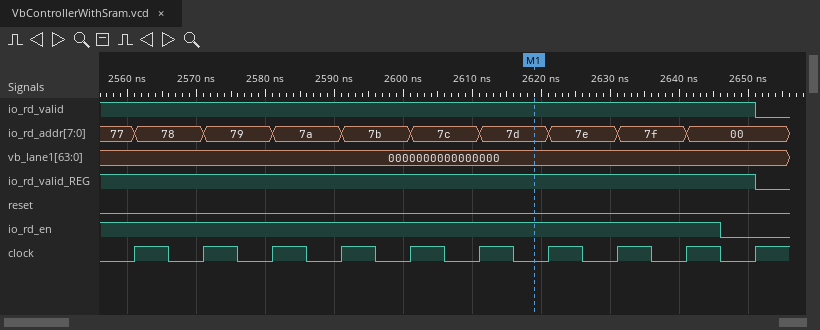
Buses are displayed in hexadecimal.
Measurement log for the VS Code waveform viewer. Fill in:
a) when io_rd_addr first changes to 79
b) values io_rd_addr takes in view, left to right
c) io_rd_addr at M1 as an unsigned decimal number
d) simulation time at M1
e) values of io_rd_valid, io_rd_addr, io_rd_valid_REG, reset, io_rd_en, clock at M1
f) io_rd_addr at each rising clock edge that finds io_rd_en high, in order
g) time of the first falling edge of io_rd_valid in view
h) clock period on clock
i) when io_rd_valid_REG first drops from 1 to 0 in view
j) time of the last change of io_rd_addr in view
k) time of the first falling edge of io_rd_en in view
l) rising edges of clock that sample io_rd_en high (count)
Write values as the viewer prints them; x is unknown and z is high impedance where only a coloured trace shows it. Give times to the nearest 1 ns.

2571 ns
77, 78, 79, 7a, 7b, 7c, 7d, 7e, 7f, 00
125
2619 ns
io_rd_valid=1, io_rd_addr=7d, io_rd_valid_REG=1, reset=0, io_rd_en=1, clock=0
77, 78, 79, 7a, 7b, 7c, 7d, 7e, 7f
2651 ns
10 ns
2651 ns
2641 ns
2646 ns
9
